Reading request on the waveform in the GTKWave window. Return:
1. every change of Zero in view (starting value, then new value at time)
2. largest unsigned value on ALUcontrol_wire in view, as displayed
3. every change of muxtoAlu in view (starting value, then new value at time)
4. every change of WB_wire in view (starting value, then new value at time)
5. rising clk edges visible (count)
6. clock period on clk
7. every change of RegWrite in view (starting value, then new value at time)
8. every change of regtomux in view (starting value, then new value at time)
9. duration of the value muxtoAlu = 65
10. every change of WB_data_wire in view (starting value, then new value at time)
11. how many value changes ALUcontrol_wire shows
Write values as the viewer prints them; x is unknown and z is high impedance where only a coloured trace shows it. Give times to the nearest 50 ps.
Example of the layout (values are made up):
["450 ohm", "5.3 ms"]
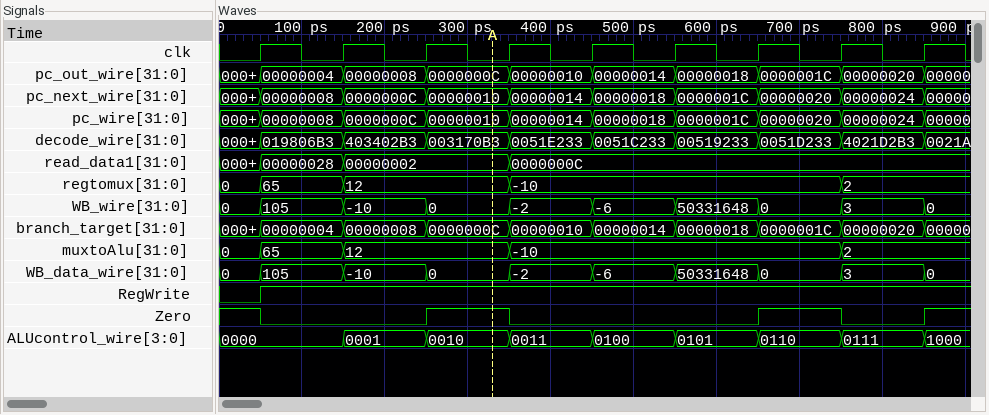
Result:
["1, 0 at 50 ps, 1 at 250 ps, 0 at 350 ps, 1 at 650 ps, 0 at 750 ps, 1 at 850 ps", "1000", "0, 65 at 50 ps, 12 at 150 ps, -10 at 350 ps, 2 at 750 ps", "0, 105 at 50 ps, -10 at 150 ps, 0 at 250 ps, -2 at 350 ps, -6 at 450 ps, 50331648 at 550 ps, 0 at 650 ps, 3 at 750 ps, 0 at 850 ps", "9", "100 ps", "0, 1 at 50 ps", "0, 65 at 50 ps, 12 at 150 ps, -10 at 350 ps, 2 at 750 ps", "100 ps", "0, 105 at 50 ps, -10 at 150 ps, 0 at 250 ps, -2 at 350 ps, -6 at 450 ps, 50331648 at 550 ps, 0 at 650 ps, 3 at 750 ps, 0 at 850 ps", "8"]
